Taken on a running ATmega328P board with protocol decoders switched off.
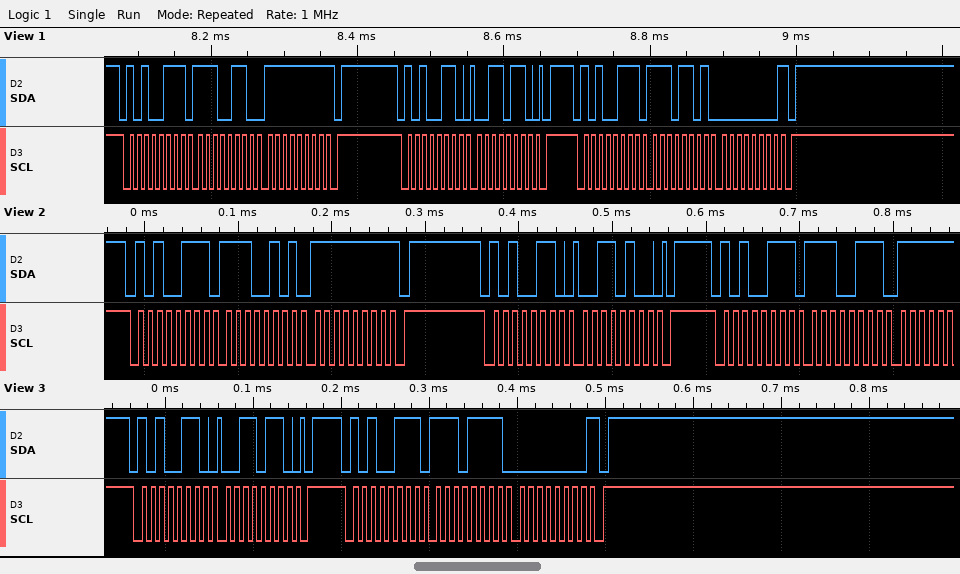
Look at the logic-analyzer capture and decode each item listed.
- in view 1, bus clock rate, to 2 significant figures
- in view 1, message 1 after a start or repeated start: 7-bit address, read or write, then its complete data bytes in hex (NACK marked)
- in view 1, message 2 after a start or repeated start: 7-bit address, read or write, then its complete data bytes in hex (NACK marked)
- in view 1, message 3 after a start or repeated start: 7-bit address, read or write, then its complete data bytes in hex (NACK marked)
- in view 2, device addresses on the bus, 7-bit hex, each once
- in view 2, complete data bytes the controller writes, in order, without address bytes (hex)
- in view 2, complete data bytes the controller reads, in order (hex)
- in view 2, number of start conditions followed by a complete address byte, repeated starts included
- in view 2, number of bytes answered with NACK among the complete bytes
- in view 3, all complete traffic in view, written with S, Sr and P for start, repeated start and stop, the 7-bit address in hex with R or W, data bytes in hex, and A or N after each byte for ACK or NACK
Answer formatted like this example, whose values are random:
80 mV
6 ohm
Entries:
100 kHz
0x53 read: E6 FF NACK
0x53 write: 36
0x53 read: ED 00 NACK
0x53
34
E5 FF E7
3
1
S 53W A 36 A P S 53R A EF A 00 N P
